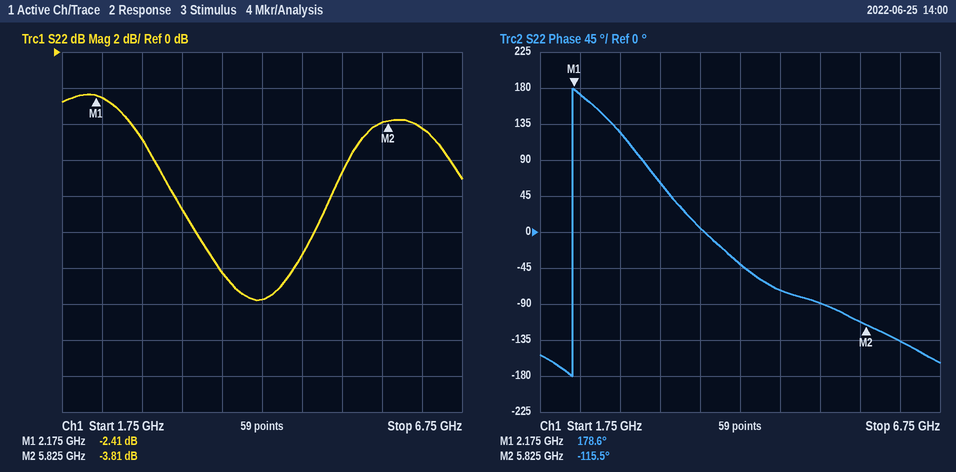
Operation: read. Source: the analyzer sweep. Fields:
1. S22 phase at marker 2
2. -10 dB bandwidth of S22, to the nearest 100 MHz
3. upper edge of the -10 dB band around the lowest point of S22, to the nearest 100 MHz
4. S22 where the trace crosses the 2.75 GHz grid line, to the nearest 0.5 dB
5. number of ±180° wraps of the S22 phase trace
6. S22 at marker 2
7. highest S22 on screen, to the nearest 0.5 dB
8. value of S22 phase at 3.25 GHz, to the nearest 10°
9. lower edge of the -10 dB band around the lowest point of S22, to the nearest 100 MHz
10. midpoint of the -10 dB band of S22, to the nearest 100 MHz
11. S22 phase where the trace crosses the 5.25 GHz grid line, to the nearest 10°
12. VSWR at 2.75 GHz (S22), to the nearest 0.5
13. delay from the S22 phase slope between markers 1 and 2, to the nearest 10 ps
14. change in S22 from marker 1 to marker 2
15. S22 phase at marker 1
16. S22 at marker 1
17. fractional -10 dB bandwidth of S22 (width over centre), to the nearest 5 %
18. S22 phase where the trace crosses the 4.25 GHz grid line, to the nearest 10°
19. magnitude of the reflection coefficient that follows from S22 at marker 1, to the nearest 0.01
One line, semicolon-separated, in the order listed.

-115.5°; 1.5 GHz; 4.9 GHz; -5.0 dB; 1; -3.81 dB; -2.5 dB; 60°; 3.4 GHz; 4.2 GHz; -90°; 3.5; 220 ps; -1.40 dB; 178.6°; -2.41 dB; 35 %; -40°; 0.76
